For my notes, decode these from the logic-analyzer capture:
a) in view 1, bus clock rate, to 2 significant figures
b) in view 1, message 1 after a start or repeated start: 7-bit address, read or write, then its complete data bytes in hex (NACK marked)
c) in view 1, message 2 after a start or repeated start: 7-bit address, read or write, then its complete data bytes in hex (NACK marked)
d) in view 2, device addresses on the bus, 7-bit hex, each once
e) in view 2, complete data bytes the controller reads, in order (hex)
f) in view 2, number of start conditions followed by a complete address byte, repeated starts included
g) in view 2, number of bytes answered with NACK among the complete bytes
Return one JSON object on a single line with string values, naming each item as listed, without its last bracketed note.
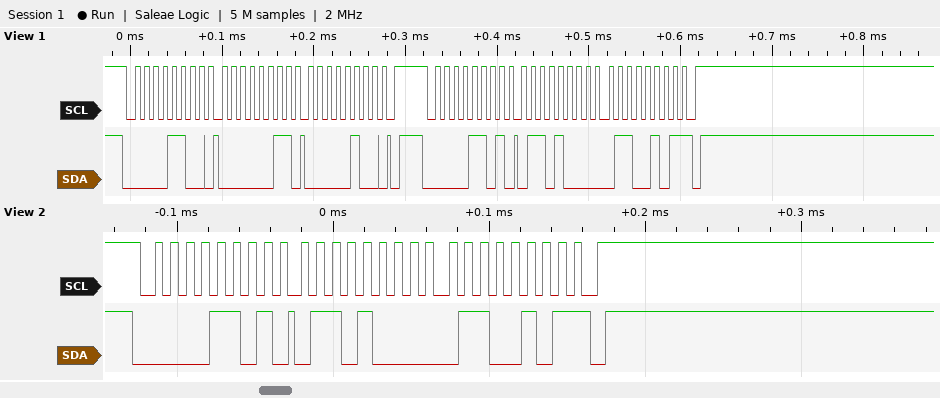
{"in view 1, bus clock rate, to 2 significant figures": "100 kHz", "in view 1, message 1 after a start or repeated start: 7-bit address, read or write, then its complete data bytes in hex": "0x06 write: 03 04", "in view 1, message 2 after a start or repeated start: 7-bit address, read or write, then its complete data bytes in hex": "0x06 read: 68 65 NACK", "in view 2, device addresses on the bus, 7-bit hex, each once": "0x06", "in view 2, complete data bytes the controller reads, in order": "68 65", "in view 2, number of start conditions followed by a complete address byte, repeated starts included": "1", "in view 2, number of bytes answered with NACK among the complete bytes": "1"}
